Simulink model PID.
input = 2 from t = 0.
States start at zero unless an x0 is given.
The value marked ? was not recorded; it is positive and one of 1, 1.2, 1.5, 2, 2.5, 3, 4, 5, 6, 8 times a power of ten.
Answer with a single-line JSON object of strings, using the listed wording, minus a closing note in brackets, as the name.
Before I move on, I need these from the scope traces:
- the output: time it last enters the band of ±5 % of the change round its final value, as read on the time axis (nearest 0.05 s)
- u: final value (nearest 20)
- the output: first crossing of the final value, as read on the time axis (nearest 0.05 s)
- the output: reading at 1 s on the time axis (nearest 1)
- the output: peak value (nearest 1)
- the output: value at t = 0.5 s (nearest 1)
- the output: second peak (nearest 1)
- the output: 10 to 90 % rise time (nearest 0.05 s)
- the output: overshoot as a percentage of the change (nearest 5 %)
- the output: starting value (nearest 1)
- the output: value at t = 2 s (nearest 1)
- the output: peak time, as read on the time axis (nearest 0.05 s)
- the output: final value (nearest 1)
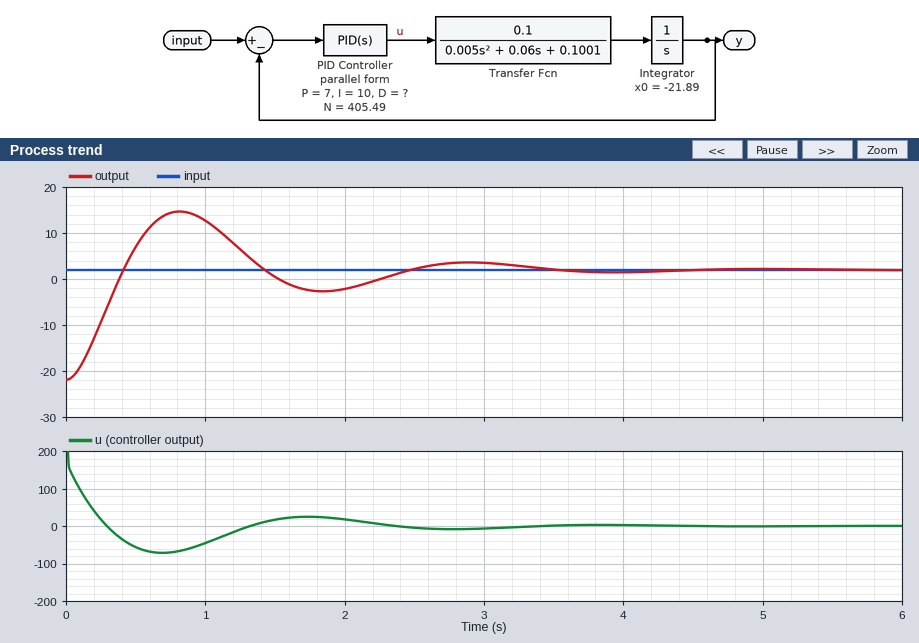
{"the output: time it last enters the band of ±5 % of the change round its final value, as read on the time axis": "3.15 s", "u: final value": "0", "the output: first crossing of the final value, as read on the time axis": "0.40 s", "the output: reading at 1 s on the time axis": "13", "the output: peak value": "15", "the output: value at t = 0.5 s": "7", "the output: second peak": "4", "the output: 10 to 90 % rise time": "0.30 s", "the output: overshoot as a percentage of the change": "55 %", "the output: starting value": "-22", "the output: value at t = 2 s": "-2", "the output: peak time, as read on the time axis": "0.80 s", "the output: final value": "2"}
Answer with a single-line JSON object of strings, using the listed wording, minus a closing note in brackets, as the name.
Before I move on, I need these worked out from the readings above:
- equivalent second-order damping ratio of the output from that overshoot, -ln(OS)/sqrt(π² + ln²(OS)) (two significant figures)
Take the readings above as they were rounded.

{"equivalent second-order damping ratio of the output from that overshoot, -ln(OS)/sqrt(π² + ln²(OS))": "0.19"}
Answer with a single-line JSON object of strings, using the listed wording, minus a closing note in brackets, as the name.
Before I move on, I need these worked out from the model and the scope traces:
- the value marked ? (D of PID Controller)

{"the value marked ?": "1.5"}
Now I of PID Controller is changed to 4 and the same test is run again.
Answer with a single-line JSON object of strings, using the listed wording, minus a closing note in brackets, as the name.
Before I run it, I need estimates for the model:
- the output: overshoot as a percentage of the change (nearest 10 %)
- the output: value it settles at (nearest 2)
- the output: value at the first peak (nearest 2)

{"the output: overshoot as a percentage of the change": "40 %", "the output: value it settles at": "2", "the output: value at the first peak": "10"}
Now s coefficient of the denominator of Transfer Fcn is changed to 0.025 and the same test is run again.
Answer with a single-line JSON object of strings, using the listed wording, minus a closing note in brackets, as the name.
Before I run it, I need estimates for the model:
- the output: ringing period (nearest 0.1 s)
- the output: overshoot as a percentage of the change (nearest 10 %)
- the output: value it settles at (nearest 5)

{"the output: ringing period": "1.0 s", "the output: overshoot as a percentage of the change": "60 %", "the output: value it settles at": "0"}
